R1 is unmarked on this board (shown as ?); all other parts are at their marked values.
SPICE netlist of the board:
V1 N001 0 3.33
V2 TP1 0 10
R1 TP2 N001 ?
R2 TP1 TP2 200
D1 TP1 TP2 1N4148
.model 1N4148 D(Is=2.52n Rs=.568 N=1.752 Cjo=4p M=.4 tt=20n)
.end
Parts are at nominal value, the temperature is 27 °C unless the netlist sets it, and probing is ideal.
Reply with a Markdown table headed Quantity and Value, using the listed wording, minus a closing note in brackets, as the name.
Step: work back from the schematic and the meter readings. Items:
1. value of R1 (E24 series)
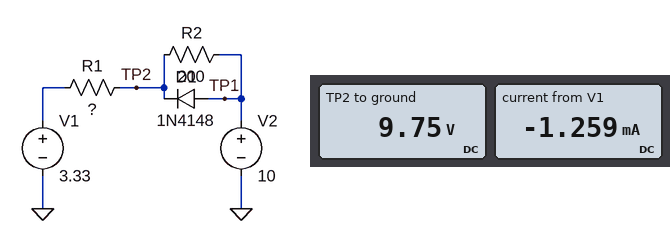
| Quantity | Value |
|---|---|
| value of R1 | 5.1 kΩ |
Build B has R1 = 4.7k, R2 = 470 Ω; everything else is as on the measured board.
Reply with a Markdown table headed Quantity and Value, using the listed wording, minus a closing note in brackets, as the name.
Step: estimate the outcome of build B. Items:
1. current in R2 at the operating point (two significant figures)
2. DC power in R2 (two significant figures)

| Quantity | Value |
|---|---|
| current in R2 at the operating point | 1.1 mA |
| DC power in R2 | 560 µW |
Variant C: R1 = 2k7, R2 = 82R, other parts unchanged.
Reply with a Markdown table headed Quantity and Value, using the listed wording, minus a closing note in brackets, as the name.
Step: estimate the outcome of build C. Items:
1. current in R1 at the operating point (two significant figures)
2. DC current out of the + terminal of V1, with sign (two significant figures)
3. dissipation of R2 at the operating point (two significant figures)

| Quantity | Value |
|---|---|
| current in R1 at the operating point | 2.4 mA |
| DC current out of the + terminal of V1, with sign | -2.4 mA |
| dissipation of R2 at the operating point | 470 µW |
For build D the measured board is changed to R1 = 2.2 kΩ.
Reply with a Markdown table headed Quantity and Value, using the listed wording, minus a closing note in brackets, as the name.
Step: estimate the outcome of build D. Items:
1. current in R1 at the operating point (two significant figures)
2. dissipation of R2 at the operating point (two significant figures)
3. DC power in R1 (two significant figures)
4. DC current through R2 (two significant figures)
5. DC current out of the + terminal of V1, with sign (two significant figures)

| Quantity | Value |
|---|---|
| current in R1 at the operating point | 2.8 mA |
| dissipation of R2 at the operating point | 1.3 mW |
| DC power in R1 | 17 mW |
| DC current through R2 | 2.6 mA |
| DC current out of the + terminal of V1, with sign | -2.8 mA |
